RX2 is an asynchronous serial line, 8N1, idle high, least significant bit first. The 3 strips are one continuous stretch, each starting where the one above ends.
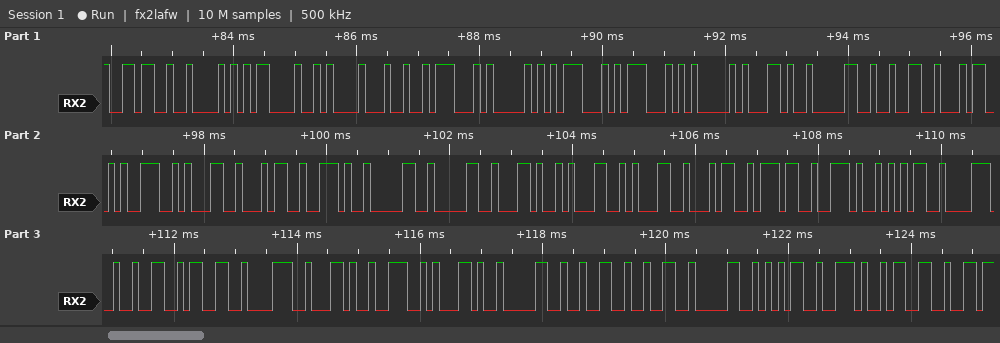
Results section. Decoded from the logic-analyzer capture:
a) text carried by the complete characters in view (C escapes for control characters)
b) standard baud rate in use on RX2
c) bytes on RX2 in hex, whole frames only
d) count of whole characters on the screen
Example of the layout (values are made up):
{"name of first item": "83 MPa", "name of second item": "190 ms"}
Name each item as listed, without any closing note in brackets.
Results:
{"text carried by the complete characters in view": "\"6B\\r\\n$GPGGA,024914.00,1147.58238,N,02205.3\"", "standard baud rate in use on RX2": "9600 baud", "bytes on RX2 in hex, whole frames only": "36 42 0D 0A 24 47 50 47 47 41 2C 30 32 34 39 31 34 2E 30 30 2C 31 31 34 37 2E 35 38 32 33 38 2C 4E 2C 30 32 32 30 35 2E 33", "count of whole characters on the screen": "41"}
